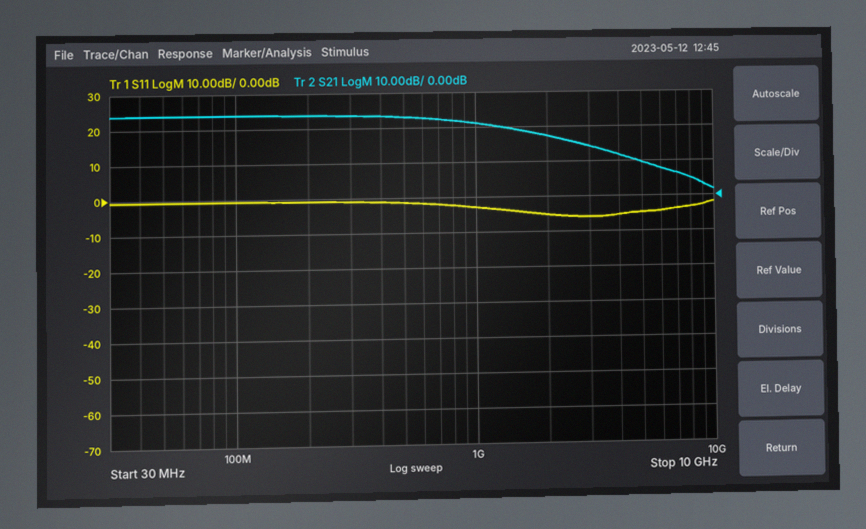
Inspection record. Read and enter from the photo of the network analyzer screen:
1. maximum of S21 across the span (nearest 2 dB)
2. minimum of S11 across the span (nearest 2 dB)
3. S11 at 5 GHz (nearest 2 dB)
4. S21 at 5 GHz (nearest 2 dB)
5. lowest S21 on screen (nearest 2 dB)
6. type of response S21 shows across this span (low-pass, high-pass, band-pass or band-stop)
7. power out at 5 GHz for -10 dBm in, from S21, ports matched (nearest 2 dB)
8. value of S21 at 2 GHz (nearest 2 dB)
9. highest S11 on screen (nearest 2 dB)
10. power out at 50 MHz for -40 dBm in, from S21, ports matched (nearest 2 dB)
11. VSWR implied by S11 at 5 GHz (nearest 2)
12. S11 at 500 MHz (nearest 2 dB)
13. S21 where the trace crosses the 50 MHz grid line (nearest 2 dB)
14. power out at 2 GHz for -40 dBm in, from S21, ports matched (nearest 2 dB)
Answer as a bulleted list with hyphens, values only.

- 24 dB
- -6 dB
- -4 dB
- 10 dB
- 2 dB
- low-pass
- 0 dBm
- 18 dB
- 0 dB
- -16 dBm
- 4
- -2 dB
- 24 dB
- -22 dBm
